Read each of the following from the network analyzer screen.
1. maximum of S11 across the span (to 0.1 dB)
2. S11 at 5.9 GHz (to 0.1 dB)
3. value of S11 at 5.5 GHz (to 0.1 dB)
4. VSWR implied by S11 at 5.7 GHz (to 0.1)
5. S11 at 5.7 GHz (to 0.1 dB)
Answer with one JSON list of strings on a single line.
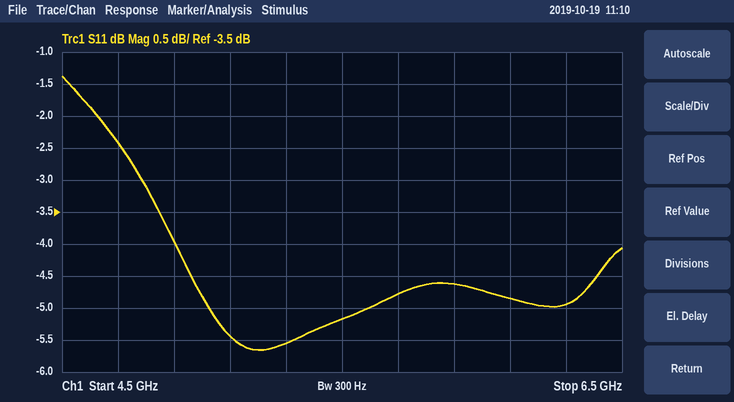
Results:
["-1.4 dB", "-4.6 dB", "-5.2 dB", "3.7", "-4.8 dB"]
